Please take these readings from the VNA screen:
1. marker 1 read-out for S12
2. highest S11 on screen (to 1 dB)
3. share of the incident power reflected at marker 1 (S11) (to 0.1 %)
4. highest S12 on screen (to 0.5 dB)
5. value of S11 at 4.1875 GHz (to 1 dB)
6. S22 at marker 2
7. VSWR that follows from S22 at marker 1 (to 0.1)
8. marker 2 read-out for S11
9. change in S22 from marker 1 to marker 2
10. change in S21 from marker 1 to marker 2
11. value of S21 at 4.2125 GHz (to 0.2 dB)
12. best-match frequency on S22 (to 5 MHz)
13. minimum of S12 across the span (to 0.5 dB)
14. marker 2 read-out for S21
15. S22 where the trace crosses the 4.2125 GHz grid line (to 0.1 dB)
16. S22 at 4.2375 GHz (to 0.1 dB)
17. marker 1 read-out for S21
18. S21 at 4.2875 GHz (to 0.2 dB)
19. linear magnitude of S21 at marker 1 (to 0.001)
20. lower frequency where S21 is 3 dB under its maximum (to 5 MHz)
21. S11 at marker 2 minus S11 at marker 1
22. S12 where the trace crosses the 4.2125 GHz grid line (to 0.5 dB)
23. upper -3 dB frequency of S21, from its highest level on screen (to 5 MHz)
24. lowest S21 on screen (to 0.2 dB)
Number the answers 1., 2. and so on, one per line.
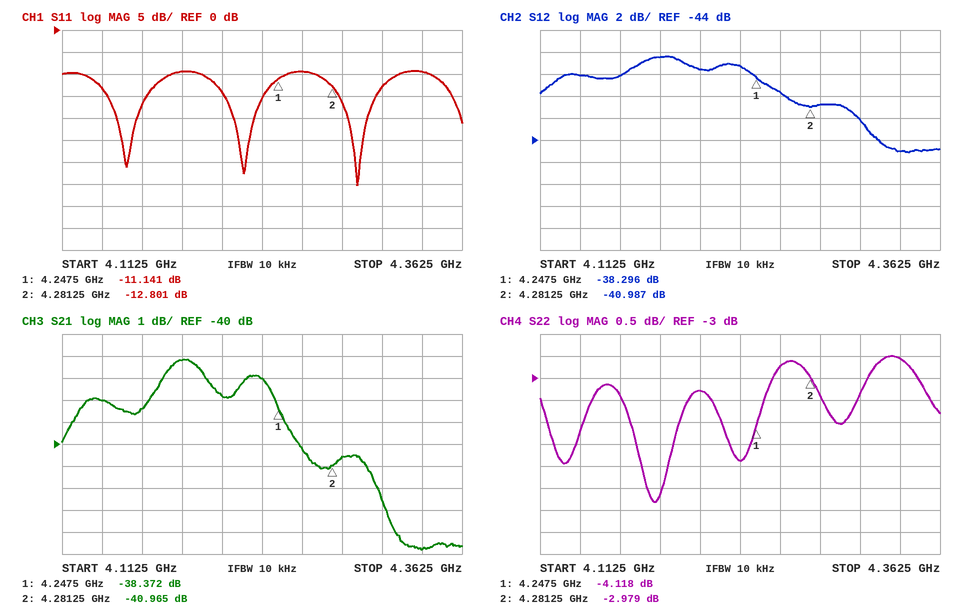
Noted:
1. -38.296 dB
2. -9 dB
3. 7.7 %
4. -36.5 dB
5. -9 dB
6. -2.979 dB
7. 4.3
8. -12.801 dB
9. 1.139 dB
10. -2.593 dB
11. -37.8 dB
12. 4.185 GHz
13. -45.0 dB
14. -40.965 dB
15. -3.3 dB
16. -4.9 dB
17. -38.372 dB
18. -40.6 dB
19. 0.012
20. 4.120 GHz
21. -1.660 dB
22. -37.5 dB
23. 4.255 GHz
24. -44.8 dB
